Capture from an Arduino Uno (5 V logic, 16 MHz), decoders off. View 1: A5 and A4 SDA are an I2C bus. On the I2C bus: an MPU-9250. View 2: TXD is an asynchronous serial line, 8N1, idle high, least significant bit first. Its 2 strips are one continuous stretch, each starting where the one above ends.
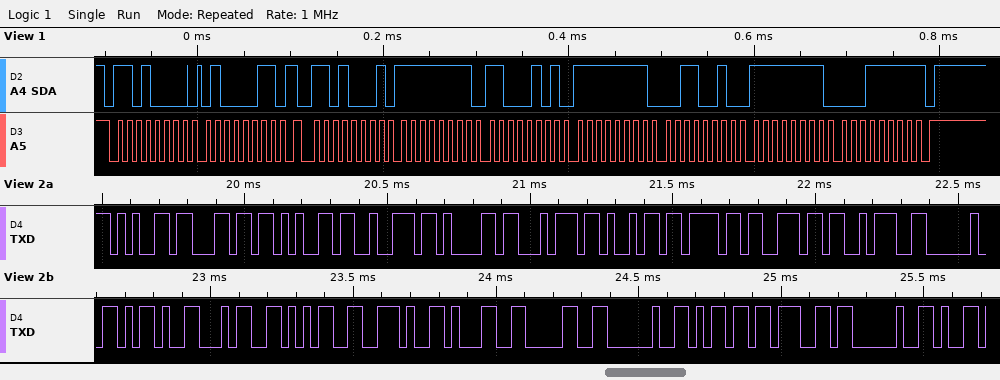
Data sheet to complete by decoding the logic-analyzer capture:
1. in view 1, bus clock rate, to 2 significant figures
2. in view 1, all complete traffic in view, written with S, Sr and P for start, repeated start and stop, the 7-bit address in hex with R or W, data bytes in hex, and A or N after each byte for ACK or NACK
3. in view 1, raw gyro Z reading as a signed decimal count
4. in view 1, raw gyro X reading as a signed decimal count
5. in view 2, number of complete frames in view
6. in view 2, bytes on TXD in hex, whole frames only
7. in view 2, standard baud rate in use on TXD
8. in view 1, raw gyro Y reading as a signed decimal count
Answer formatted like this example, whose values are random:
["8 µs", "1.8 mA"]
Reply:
["100 kHz", "S 68W A 43 A Sr 68R A FF A C5 A FF A 32 A FF A 1F N P", "-225", "-59", "21", "65 6C 65 72 61 74 69 6F 6E 3A 20 2D 34 35 2E 31 30 20 6D 67 20", "38400 baud", "-206"]
